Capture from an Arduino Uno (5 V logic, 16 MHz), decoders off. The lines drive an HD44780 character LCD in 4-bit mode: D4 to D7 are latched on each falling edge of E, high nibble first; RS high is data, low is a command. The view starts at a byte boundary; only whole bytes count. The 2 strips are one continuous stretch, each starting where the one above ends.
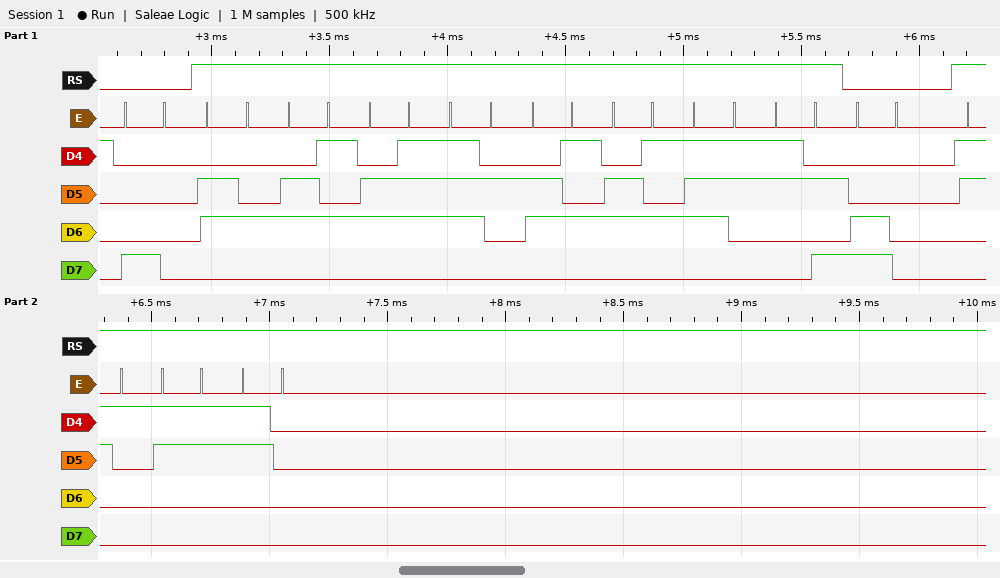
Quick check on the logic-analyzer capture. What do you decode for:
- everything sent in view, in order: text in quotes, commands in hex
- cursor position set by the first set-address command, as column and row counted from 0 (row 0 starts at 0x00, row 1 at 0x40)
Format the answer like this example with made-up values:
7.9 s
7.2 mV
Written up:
0x80 "degrees:" 0xC0 "130"
column 0, row 0
